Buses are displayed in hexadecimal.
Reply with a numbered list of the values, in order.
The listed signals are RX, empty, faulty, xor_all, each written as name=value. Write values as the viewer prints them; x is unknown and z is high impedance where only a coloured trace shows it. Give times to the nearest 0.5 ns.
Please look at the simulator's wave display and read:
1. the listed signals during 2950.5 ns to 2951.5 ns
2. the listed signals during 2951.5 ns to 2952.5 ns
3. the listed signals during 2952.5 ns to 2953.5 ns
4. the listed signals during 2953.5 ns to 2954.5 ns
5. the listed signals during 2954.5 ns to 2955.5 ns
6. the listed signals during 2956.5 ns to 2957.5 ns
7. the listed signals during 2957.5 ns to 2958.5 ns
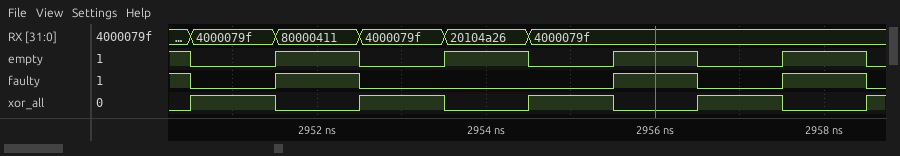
1. RX=4000079f, empty=0, faulty=0, xor_all=1
2. RX=80000411, empty=1, faulty=1, xor_all=0
3. RX=4000079f, empty=0, faulty=0, xor_all=1
4. RX=20104a26, empty=1, faulty=0, xor_all=0
5. RX=4000079f, empty=0, faulty=0, xor_all=1
6. RX=4000079f, empty=0, faulty=0, xor_all=1
7. RX=4000079f, empty=1, faulty=1, xor_all=0
